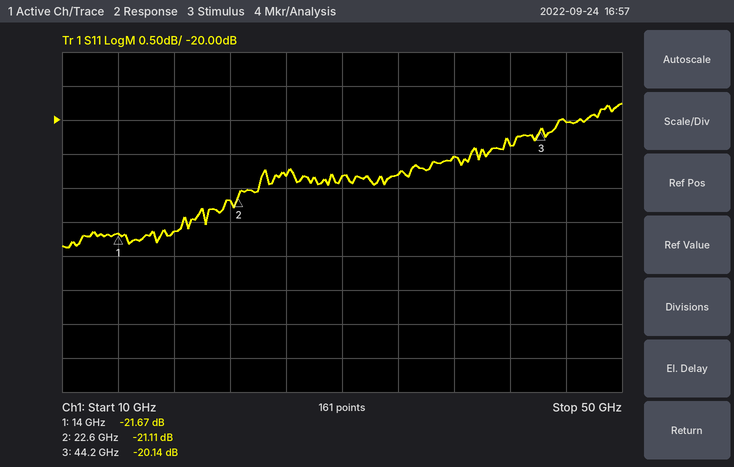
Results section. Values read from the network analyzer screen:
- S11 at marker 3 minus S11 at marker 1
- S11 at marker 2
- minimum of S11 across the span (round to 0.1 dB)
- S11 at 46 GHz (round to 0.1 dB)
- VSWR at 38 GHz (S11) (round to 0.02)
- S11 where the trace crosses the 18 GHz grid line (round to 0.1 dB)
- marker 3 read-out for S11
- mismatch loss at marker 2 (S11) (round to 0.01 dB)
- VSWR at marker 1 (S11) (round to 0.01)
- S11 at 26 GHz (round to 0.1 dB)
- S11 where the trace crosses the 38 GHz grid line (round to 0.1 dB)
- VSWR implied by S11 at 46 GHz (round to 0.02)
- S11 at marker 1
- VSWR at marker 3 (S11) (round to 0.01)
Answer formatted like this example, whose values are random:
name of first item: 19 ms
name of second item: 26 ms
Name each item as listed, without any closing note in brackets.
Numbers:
S11 at marker 3 minus S11 at marker 1: 1.53 dB
S11 at marker 2: -21.11 dB
minimum of S11 across the span: -21.9 dB
S11 at 46 GHz: -20.0 dB
VSWR at 38 GHz (S11): 1.20
S11 where the trace crosses the 18 GHz grid line: -21.6 dB
marker 3 read-out for S11: -20.14 dB
mismatch loss at marker 2 (S11): 0.03 dB
VSWR at marker 1 (S11): 1.18
S11 at 26 GHz: -20.8 dB
S11 where the trace crosses the 38 GHz grid line: -20.5 dB
VSWR implied by S11 at 46 GHz: 1.22
S11 at marker 1: -21.67 dB
VSWR at marker 3 (S11): 1.22
